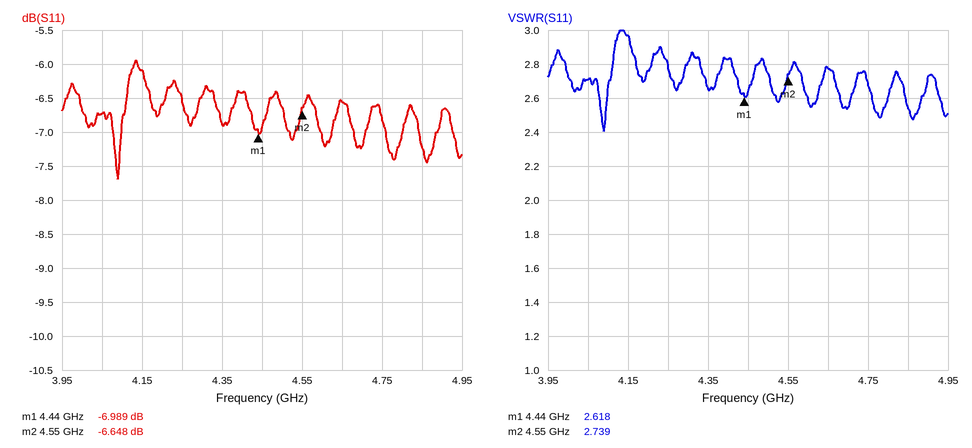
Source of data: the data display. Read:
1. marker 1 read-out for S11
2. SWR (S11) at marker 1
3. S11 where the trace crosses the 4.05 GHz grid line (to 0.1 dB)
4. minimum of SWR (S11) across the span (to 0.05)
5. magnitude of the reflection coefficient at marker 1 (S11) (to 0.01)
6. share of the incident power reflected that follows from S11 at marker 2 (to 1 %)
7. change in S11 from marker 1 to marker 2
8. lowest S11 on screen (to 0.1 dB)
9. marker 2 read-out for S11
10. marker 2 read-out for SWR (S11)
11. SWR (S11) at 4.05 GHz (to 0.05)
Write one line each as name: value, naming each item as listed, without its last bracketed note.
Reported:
marker 1 read-out for S11: -6.989 dB
SWR (S11) at marker 1: 2.618
S11 where the trace crosses the 4.05 GHz grid line: -6.7 dB
minimum of SWR (S11) across the span: 2.40
magnitude of the reflection coefficient at marker 1 (S11): 0.45
share of the incident power reflected that follows from S11 at marker 2: 22 %
change in S11 from marker 1 to marker 2: 0.341 dB
lowest S11 on screen: -7.7 dB
marker 2 read-out for S11: -6.648 dB
marker 2 read-out for SWR: 2.739
SWR (S11) at 4.05 GHz: 2.70
